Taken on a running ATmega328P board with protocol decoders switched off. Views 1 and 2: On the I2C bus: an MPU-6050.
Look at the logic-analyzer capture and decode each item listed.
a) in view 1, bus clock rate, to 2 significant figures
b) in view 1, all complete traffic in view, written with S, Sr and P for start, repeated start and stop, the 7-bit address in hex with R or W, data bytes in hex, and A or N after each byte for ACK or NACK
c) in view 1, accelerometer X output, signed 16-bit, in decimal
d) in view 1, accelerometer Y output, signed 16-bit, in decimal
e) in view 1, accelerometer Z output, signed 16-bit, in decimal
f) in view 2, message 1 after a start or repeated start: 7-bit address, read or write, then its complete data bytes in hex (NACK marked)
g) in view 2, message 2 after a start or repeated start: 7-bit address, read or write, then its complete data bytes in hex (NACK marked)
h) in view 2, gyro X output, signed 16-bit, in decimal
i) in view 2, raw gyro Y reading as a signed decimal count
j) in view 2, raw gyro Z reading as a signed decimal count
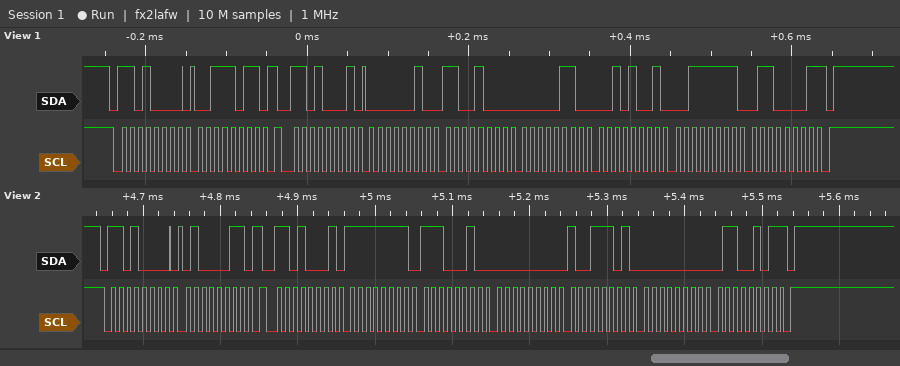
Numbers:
100 kHz
S 68W A 3B A Sr 68R A 02 A C8 A 06 A 29 A 3F A 61 N P
712
1577
16225
0x68 write: 43
0x68 read: FF E2 00 9D 00 65 NACK
-30
157
101
